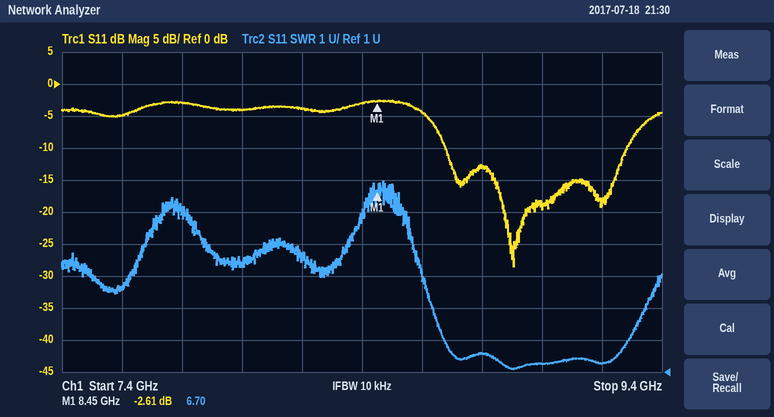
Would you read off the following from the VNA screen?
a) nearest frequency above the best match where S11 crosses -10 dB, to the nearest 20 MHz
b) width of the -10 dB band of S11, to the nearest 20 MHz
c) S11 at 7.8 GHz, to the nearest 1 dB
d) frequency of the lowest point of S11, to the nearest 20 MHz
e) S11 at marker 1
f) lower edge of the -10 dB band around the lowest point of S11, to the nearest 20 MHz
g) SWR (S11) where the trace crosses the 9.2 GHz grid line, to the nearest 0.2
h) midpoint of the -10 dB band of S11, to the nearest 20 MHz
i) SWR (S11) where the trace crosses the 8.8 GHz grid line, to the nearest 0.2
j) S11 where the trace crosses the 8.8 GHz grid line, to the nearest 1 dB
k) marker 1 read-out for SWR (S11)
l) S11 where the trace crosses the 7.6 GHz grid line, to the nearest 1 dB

9.28 GHz
600 MHz
-3 dB
8.90 GHz
-2.61 dB
8.68 GHz
1.2
8.98 GHz
1.6
-13 dB
6.70
-5 dB
